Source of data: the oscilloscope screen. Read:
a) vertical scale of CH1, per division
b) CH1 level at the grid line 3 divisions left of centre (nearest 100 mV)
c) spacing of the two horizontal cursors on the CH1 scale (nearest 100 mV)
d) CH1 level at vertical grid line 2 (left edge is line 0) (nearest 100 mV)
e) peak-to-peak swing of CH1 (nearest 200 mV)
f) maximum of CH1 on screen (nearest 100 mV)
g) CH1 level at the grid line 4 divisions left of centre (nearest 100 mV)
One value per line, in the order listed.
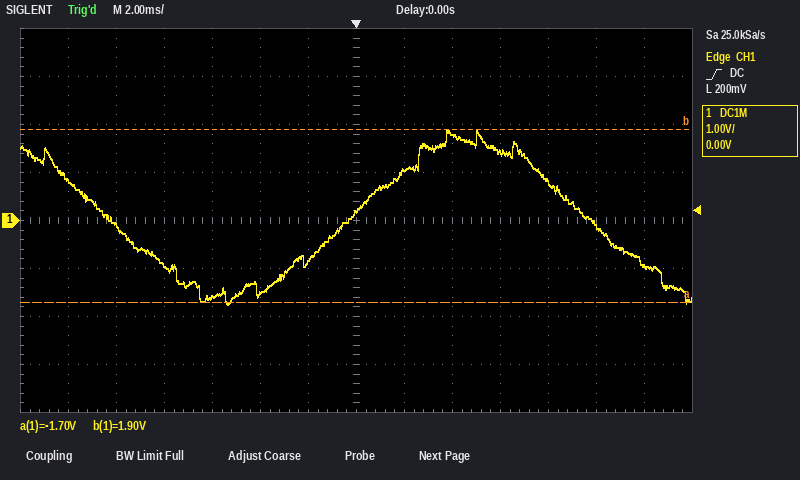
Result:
1 V
-1.6 V
3.6 V
-100 mV
3.6 V
1.9 V
-900 mV
